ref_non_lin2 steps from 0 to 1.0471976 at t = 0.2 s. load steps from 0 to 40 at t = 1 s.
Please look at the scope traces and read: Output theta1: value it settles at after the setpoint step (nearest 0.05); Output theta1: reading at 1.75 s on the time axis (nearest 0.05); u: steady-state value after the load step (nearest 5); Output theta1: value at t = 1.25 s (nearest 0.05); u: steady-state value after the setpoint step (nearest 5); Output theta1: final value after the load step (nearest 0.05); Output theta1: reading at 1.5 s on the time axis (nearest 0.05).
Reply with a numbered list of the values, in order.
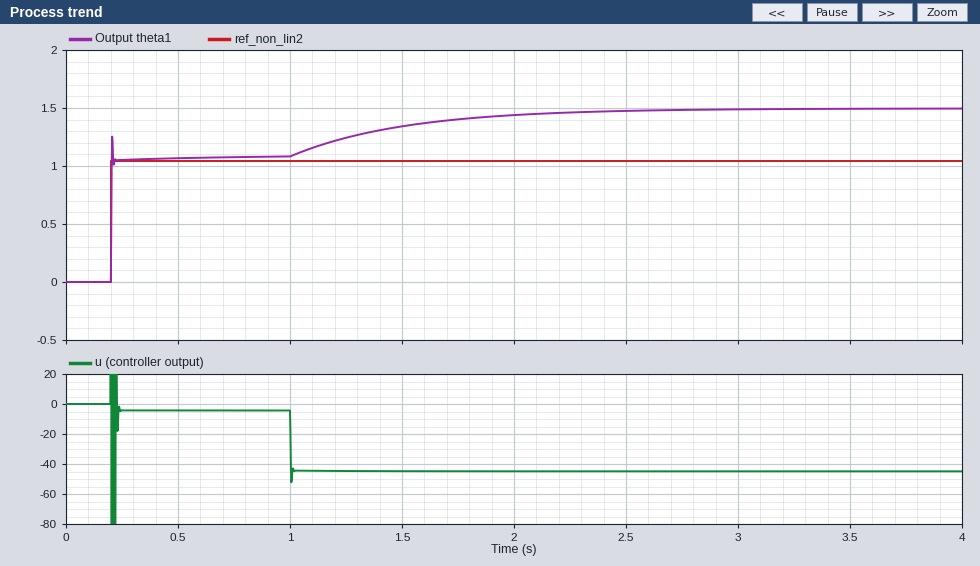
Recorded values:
1. 1.10
2. 1.40
3. -45
4. 1.25
5. -5
6. 1.50
7. 1.35
